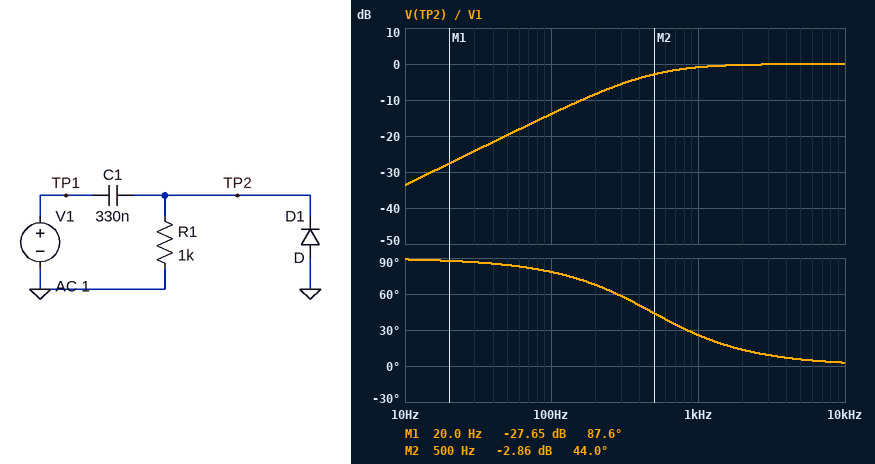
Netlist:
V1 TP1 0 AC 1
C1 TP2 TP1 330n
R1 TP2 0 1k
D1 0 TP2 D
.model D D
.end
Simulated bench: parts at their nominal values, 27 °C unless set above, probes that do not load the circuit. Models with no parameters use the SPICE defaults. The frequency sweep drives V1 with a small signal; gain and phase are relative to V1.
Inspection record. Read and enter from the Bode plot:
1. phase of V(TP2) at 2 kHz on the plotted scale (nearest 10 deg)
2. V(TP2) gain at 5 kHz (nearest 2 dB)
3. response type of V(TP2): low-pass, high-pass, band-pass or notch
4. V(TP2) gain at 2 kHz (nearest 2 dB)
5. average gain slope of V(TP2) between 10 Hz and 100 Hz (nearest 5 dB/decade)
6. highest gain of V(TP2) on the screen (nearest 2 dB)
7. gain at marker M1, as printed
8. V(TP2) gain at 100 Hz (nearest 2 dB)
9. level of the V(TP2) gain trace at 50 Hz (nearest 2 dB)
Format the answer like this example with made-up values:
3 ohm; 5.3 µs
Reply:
10 deg; 0 dB; high-pass; 0 dB; 20 dB/decade; 0 dB; -27.65 dB; -14 dB; -20 dB
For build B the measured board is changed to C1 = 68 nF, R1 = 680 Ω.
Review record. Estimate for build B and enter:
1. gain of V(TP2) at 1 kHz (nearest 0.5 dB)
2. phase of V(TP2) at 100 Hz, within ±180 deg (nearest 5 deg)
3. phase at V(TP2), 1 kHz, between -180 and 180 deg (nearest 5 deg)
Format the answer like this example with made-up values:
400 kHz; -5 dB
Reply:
-11.0 dB; 90 deg; 75 deg
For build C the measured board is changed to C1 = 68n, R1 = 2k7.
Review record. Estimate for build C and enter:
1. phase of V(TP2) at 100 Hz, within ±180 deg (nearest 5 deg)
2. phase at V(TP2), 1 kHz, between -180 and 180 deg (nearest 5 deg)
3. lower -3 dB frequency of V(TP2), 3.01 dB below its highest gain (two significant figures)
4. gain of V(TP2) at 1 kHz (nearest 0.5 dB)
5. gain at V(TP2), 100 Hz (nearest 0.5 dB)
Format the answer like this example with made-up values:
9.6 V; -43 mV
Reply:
85 deg; 40 deg; 870 Hz; -2.5 dB; -19.0 dB
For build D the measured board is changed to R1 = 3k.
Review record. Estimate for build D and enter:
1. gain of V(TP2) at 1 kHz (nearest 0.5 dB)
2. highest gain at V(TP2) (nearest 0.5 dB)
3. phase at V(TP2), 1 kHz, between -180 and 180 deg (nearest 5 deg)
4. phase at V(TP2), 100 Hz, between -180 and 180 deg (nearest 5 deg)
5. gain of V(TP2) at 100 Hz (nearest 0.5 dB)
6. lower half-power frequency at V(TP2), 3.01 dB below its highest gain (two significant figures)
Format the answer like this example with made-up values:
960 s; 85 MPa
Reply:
0 dB; 0 dB; 10 deg; 60 deg; -5.5 dB; 160 Hz
